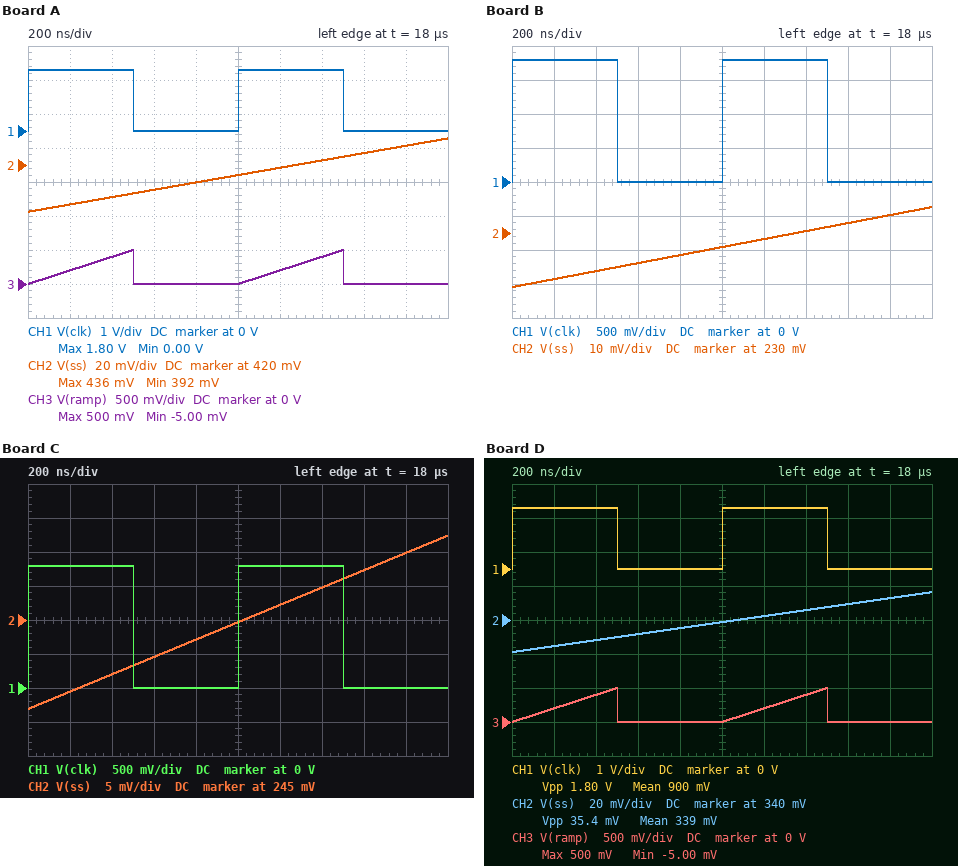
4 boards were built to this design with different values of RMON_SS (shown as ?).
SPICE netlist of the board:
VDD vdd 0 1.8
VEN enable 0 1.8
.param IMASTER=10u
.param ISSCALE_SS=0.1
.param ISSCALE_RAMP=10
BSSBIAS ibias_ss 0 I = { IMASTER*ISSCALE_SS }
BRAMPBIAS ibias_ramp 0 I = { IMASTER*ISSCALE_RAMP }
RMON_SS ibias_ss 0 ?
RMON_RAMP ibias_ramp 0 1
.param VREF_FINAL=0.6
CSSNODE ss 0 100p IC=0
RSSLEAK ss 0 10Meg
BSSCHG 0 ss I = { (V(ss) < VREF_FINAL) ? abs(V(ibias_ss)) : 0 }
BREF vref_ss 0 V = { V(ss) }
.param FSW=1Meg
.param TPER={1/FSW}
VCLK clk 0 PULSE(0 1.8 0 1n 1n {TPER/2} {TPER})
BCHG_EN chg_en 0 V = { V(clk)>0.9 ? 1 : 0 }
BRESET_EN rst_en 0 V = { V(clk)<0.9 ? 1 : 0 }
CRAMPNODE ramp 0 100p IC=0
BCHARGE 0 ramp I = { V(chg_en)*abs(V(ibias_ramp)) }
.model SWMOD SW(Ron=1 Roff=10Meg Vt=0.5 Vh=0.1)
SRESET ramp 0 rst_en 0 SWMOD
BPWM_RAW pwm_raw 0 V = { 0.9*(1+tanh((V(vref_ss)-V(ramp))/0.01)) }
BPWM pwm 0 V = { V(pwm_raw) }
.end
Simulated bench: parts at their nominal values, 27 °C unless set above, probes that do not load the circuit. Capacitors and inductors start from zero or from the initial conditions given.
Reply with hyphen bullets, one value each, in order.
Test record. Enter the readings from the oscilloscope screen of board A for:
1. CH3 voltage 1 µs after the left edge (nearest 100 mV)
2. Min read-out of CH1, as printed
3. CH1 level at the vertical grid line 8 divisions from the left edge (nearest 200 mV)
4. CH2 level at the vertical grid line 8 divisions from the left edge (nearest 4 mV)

- 0 V
- 0.00 V
- 0 V
- 428 mV
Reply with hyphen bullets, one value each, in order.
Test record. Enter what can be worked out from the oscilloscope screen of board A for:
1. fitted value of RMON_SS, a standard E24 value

- 2.2 Ω
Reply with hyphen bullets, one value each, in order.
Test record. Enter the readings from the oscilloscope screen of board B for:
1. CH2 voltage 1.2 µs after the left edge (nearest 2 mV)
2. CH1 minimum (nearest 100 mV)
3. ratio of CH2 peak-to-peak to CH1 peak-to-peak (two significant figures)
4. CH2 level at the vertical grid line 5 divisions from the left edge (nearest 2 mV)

- 228 mV
- 0 V
- 0.013
- 226 mV
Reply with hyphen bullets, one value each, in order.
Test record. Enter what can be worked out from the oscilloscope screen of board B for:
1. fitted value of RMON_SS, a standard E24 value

- 1.2 Ω
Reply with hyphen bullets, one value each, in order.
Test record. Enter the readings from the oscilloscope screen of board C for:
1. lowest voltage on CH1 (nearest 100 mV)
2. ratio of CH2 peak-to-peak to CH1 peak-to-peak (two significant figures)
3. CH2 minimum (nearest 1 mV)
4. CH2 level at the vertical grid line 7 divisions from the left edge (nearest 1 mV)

- 0 V
- 0.014
- 232 mV
- 250 mV
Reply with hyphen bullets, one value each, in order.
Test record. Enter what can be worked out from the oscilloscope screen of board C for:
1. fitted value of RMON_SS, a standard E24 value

- 1.3 Ω
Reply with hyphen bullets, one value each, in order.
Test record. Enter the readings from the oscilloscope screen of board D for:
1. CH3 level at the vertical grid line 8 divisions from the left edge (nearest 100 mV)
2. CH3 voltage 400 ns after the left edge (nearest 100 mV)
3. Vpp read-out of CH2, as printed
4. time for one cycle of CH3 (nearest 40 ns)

- 0 V
- 400 mV
- 35.4 mV
- 1.00 µs
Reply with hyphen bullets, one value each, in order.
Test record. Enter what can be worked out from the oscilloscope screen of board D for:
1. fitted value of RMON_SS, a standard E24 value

- 1.8 Ω
